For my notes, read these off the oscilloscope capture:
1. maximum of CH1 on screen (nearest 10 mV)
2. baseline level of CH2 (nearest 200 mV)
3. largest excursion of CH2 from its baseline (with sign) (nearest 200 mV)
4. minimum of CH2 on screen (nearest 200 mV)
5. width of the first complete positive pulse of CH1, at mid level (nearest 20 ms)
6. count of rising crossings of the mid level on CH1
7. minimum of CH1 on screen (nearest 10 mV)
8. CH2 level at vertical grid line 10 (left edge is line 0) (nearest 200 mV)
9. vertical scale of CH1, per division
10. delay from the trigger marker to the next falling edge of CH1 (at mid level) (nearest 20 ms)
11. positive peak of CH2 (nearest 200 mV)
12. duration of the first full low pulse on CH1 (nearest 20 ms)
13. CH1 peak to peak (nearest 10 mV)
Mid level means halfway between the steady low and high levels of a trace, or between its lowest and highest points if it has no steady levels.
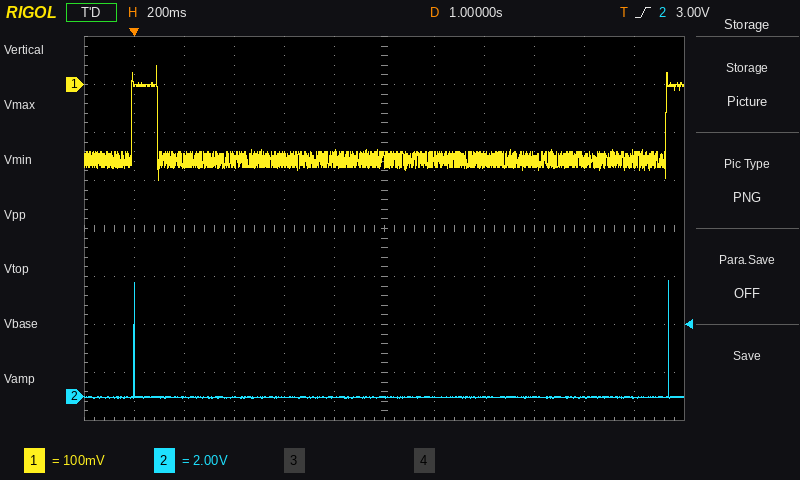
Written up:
40 mV
0.0 V
+4.8 V
0.0 V
100 ms
2
-200 mV
0.0 V
100 mV
100 ms
4.8 V
2.04 s
240 mV
